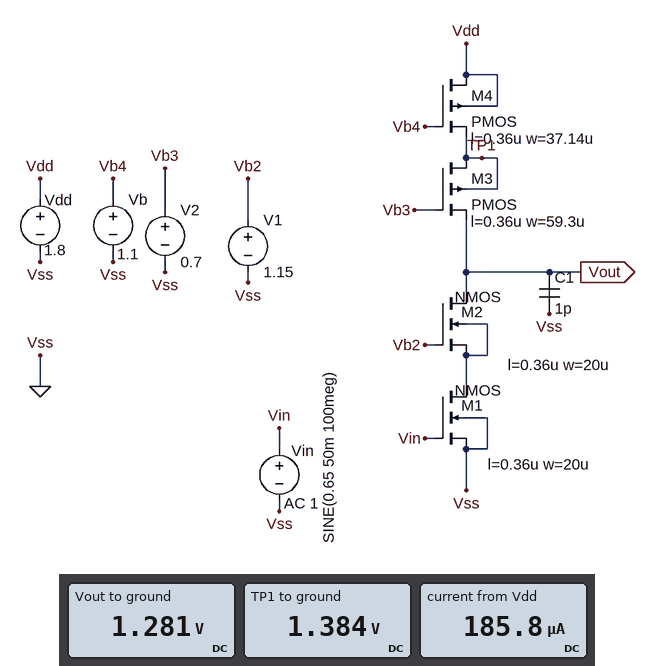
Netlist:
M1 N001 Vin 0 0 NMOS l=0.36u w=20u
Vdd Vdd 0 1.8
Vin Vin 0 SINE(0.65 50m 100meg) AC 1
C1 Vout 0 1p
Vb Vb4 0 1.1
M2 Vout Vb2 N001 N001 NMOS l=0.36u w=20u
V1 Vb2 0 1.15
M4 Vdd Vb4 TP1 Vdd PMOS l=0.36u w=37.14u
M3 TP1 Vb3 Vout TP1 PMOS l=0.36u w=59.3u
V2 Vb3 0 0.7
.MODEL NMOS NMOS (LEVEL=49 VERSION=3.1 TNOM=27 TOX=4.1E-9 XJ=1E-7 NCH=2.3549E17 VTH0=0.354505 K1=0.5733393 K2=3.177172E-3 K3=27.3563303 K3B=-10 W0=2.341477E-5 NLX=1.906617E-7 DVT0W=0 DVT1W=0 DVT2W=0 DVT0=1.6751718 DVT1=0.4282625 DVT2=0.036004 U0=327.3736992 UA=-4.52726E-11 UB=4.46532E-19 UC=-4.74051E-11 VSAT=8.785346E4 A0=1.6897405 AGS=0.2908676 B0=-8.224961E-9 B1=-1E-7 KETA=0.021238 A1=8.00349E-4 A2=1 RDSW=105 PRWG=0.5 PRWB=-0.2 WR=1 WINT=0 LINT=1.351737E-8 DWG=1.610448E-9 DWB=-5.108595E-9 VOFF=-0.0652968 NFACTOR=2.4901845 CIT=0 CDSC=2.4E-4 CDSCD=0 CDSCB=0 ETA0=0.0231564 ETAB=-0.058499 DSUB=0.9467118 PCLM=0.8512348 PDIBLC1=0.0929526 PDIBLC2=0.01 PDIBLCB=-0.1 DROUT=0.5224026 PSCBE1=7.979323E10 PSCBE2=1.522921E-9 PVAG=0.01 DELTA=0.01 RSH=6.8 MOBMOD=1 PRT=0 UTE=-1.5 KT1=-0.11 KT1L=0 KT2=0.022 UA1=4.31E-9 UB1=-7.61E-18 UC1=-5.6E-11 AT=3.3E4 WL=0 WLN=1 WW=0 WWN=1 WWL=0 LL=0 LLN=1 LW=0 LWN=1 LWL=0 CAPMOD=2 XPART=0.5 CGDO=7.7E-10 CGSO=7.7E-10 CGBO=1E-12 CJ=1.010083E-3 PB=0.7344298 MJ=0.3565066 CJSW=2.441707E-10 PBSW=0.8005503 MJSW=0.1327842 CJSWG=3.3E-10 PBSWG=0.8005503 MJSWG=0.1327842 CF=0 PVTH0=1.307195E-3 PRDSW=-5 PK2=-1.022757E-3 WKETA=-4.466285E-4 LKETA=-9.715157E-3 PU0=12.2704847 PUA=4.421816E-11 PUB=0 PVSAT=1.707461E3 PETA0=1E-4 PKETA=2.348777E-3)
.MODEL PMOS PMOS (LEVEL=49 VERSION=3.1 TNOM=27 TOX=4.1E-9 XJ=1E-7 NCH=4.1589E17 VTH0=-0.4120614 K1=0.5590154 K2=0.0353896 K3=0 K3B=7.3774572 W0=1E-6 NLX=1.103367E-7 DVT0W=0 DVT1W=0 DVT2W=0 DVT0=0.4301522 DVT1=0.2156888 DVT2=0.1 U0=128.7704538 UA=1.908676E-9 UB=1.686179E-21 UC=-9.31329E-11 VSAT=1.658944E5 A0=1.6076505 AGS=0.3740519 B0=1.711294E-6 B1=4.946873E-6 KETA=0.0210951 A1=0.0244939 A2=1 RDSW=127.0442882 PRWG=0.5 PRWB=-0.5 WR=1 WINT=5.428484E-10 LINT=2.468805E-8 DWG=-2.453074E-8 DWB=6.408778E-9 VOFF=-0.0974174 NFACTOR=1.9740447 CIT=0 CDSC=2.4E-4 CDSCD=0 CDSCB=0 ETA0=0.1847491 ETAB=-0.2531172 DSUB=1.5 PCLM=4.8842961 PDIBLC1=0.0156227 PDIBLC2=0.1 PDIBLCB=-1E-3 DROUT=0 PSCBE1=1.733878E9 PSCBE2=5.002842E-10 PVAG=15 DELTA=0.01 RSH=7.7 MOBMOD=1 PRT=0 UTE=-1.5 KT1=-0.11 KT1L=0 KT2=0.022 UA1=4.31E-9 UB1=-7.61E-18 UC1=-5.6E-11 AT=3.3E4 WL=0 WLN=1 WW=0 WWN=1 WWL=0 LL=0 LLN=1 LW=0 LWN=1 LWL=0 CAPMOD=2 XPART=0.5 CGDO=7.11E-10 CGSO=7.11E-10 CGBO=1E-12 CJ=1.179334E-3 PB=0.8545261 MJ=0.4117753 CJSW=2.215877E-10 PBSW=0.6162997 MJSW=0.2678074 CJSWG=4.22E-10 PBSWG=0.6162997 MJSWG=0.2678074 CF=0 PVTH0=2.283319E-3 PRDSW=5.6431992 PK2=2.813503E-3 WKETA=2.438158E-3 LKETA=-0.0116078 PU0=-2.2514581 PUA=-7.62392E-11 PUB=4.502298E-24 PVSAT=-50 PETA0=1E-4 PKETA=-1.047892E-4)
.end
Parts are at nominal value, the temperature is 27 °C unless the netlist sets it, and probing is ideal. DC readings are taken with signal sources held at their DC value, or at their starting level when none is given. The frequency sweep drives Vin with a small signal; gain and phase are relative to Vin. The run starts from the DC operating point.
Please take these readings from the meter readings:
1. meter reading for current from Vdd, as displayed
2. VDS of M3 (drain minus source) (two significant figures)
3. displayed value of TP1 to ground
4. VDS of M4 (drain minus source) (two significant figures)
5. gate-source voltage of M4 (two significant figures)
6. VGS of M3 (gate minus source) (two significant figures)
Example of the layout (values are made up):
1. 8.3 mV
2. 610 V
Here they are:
1. 185.8 µA
2. 100 mV
3. 1.384 V
4. 420 mV
5. -280 mV
6. -580 mV
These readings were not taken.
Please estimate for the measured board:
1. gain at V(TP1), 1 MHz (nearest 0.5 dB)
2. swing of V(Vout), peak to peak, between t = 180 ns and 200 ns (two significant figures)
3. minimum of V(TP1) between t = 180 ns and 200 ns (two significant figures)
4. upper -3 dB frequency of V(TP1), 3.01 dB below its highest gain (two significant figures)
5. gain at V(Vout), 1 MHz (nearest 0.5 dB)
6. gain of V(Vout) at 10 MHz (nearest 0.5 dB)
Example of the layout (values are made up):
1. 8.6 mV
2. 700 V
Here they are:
1. 39.0 dB
2. 300 mV
3. 1.3 V
4. 1.3 MHz
5. 45.0 dB
6. 29.5 dB
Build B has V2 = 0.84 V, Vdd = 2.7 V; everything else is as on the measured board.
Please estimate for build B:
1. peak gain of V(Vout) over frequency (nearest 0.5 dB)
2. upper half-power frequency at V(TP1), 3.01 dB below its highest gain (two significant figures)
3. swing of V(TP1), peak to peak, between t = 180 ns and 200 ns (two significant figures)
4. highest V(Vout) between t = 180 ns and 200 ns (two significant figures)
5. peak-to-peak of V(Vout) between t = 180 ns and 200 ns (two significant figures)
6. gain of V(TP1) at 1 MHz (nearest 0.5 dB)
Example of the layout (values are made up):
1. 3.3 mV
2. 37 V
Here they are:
1. -5.0 dB
2. 500 MHz
3. 35 mV
4. 2.7 V
5. 56 mV
6. -9.0 dB
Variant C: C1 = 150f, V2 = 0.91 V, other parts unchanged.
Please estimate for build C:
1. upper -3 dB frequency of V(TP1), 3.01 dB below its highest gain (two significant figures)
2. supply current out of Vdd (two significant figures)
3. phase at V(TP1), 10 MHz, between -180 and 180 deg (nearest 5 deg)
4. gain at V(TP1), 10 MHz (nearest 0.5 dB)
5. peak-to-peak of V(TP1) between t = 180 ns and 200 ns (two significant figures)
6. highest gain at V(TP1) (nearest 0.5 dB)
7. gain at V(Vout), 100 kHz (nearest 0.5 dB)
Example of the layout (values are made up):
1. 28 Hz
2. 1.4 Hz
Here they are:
1. 18 MHz
2. 180 µA
3. 155 deg
4. -7.0 dB
5. 18 mV
6. -6.0 dB
7. 36.5 dB
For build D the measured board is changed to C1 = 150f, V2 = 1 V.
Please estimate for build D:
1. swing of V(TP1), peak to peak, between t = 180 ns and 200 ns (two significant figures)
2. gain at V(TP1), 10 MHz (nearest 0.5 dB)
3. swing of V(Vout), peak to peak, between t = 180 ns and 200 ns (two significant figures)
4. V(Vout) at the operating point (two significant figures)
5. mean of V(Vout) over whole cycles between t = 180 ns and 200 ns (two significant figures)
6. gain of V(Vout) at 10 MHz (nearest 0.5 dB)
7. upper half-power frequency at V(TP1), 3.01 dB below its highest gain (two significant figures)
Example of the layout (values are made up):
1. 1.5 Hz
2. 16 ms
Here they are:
1. 10 mV
2. -25.0 dB
3. 980 mV
4. 180 mV
5. 490 mV
6. 19.0 dB
7. 1.6 GHz
